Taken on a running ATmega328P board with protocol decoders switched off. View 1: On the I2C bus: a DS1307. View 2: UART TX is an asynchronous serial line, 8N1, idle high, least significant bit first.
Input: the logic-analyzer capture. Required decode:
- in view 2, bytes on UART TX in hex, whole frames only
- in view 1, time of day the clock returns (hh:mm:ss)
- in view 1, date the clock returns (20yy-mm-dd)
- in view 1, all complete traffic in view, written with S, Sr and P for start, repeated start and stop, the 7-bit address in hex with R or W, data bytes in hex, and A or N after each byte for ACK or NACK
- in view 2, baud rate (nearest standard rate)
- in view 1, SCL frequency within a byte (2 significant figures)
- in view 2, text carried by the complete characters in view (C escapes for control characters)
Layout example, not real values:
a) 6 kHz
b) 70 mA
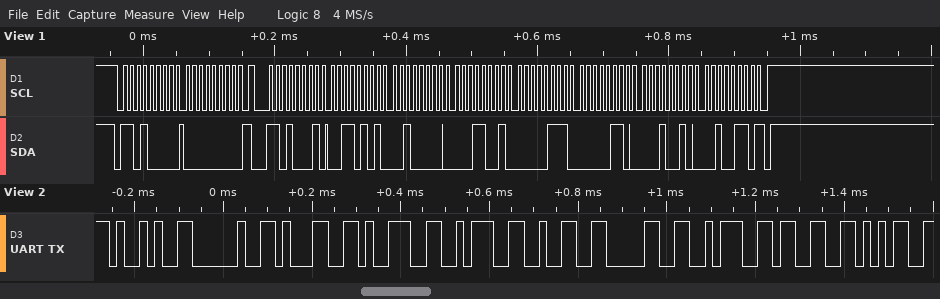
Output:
a) 29 20 31 39 3A 32 30 3A 33 35
b) 19:20:35
c) 2026-12-06
d) S 68W A 00 A Sr 68R A 35 A 20 A 19 A 07 A 06 A 12 A 26 N P
e) 57600 baud
f) 100 kHz
g) ") 19:20:35"
